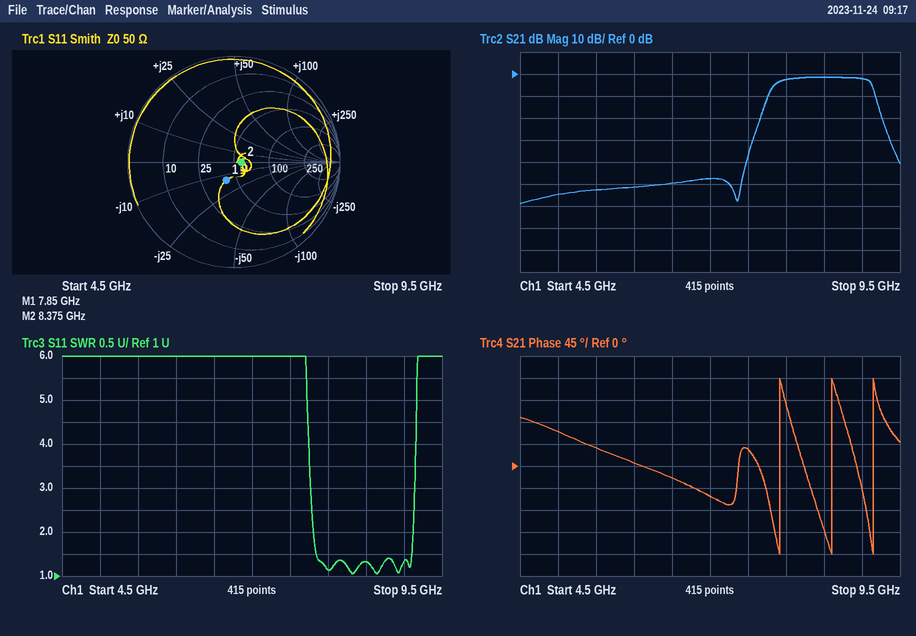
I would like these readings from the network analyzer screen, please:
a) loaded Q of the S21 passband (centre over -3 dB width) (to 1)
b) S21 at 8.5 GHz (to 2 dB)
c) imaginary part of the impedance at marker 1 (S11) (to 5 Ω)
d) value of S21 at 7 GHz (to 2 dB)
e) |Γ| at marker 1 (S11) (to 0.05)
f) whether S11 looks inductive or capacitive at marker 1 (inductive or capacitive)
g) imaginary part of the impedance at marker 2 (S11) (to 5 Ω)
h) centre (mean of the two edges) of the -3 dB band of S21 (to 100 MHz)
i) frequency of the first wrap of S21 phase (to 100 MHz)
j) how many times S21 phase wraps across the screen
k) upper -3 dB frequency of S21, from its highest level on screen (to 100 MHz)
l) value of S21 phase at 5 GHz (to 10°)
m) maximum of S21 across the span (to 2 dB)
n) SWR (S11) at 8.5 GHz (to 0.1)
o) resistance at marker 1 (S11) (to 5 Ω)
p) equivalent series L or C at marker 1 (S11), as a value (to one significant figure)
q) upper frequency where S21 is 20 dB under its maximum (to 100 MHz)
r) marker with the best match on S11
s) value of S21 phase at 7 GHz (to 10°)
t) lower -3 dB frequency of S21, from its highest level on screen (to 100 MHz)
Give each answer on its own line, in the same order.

7
-2 dB
-15 Ω
-48 dB
0.20
capacitive
0 Ω
8.5 GHz
7.9 GHz
3
9.1 GHz
70°
-2 dB
1.3
40 Ω
1 pF
9.3 GHz
marker 2
-60°
7.9 GHz
